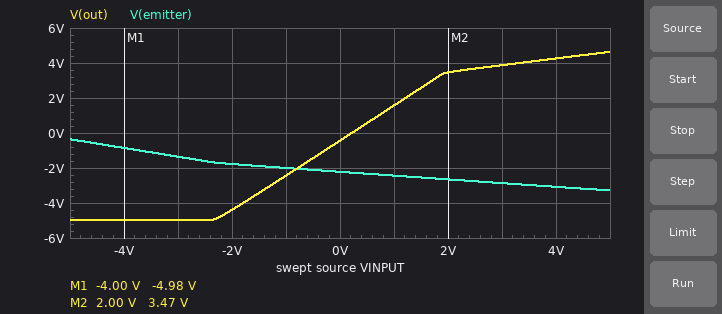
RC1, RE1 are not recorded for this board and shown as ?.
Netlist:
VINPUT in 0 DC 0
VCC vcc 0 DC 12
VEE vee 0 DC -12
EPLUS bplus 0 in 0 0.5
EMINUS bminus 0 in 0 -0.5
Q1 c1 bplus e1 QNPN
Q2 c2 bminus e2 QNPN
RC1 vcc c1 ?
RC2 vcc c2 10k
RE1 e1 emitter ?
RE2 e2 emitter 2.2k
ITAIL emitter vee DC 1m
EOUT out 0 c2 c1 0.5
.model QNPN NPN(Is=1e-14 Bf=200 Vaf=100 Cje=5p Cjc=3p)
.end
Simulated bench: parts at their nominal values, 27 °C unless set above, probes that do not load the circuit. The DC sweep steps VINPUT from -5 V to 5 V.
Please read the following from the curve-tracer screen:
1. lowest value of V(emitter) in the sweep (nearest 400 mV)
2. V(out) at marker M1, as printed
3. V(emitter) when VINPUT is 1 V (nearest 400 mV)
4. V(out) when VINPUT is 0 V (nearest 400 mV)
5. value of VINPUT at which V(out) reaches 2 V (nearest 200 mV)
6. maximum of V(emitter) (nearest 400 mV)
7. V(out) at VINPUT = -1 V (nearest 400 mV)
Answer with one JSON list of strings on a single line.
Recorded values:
["-3.2 V", "-4.98 V", "-2.4 V", "-400 mV", "1.2 V", "-400 mV", "-2.4 V"]
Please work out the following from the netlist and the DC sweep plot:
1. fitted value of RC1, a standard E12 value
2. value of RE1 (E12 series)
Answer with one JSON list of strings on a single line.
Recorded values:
["22 kΩ", "5.6 kΩ"]
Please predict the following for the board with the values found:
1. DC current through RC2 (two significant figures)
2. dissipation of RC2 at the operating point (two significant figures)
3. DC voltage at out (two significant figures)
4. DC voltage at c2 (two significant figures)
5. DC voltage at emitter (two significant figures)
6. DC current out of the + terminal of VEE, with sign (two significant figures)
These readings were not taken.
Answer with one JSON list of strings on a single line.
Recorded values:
["710 µA", "5.1 mW", "-440 mV", "4.9 V", "-2.2 V", "-1.0 mA"]
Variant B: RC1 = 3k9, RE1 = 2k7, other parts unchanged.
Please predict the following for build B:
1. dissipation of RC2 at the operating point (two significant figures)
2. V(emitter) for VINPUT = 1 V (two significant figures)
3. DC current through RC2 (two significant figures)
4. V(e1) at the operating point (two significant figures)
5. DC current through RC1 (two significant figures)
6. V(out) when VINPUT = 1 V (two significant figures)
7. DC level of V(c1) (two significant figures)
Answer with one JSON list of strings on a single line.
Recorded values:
["3.0 mW", "-1.9 V", "550 µA", "-630 mV", "450 µA", "-480 mV", "10 V"]
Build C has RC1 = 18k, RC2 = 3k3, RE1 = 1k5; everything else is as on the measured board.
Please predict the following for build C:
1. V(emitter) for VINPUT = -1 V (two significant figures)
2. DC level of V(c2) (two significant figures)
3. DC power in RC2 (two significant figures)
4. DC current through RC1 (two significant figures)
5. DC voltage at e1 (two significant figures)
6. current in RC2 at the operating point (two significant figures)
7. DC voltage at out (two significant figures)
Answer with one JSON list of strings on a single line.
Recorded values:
["-1.6 V", "11 V", "550 µW", "590 µA", "-640 mV", "410 µA", "4.6 V"]
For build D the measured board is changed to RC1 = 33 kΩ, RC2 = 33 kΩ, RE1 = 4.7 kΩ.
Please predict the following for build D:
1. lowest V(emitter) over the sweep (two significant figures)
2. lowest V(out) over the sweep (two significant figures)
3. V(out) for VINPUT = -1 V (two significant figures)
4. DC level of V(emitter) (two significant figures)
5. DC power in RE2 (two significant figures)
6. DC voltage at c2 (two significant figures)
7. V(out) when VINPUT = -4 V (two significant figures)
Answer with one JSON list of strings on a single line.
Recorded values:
["-2.9 V", "-5.7 V", "-3.1 V", "-2.1 V", "1.0 mW", "-620 mV", "-5.3 V"]
